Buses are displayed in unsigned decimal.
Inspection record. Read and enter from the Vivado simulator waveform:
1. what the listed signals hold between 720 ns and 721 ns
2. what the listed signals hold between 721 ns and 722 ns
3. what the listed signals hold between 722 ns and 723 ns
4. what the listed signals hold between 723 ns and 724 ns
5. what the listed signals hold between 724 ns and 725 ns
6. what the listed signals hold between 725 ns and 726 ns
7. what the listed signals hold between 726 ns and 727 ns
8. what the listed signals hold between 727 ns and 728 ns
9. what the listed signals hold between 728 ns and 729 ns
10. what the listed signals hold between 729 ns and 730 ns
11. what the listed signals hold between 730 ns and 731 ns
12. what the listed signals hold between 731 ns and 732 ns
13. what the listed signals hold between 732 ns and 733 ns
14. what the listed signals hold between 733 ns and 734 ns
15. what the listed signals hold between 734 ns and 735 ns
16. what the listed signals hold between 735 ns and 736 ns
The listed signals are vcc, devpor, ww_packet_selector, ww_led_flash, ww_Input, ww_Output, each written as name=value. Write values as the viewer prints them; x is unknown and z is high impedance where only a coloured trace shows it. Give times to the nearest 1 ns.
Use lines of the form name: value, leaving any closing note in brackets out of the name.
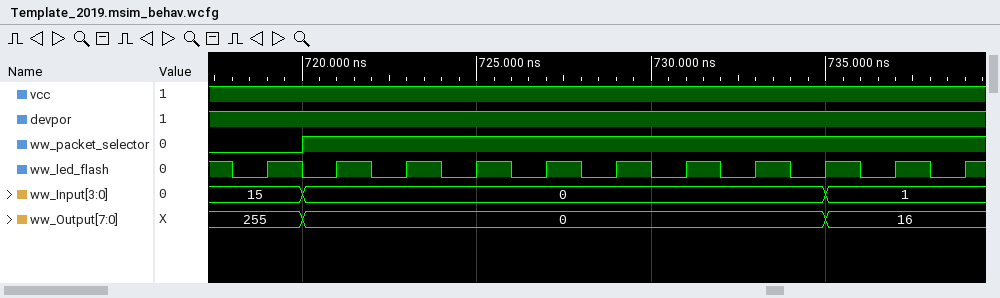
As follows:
what the listed signals hold between 720 ns and 721 ns: vcc=1, devpor=1, ww_packet_selector=1, ww_led_flash=0, ww_Input=0, ww_Output=0
what the listed signals hold between 721 ns and 722 ns: vcc=1, devpor=1, ww_packet_selector=1, ww_led_flash=1, ww_Input=0, ww_Output=0
what the listed signals hold between 722 ns and 723 ns: vcc=1, devpor=1, ww_packet_selector=1, ww_led_flash=0, ww_Input=0, ww_Output=0
what the listed signals hold between 723 ns and 724 ns: vcc=1, devpor=1, ww_packet_selector=1, ww_led_flash=1, ww_Input=0, ww_Output=0
what the listed signals hold between 724 ns and 725 ns: vcc=1, devpor=1, ww_packet_selector=1, ww_led_flash=0, ww_Input=0, ww_Output=0
what the listed signals hold between 725 ns and 726 ns: vcc=1, devpor=1, ww_packet_selector=1, ww_led_flash=1, ww_Input=0, ww_Output=0
what the listed signals hold between 726 ns and 727 ns: vcc=1, devpor=1, ww_packet_selector=1, ww_led_flash=0, ww_Input=0, ww_Output=0
what the listed signals hold between 727 ns and 728 ns: vcc=1, devpor=1, ww_packet_selector=1, ww_led_flash=1, ww_Input=0, ww_Output=0
what the listed signals hold between 728 ns and 729 ns: vcc=1, devpor=1, ww_packet_selector=1, ww_led_flash=0, ww_Input=0, ww_Output=0
what the listed signals hold between 729 ns and 730 ns: vcc=1, devpor=1, ww_packet_selector=1, ww_led_flash=1, ww_Input=0, ww_Output=0
what the listed signals hold between 730 ns and 731 ns: vcc=1, devpor=1, ww_packet_selector=1, ww_led_flash=0, ww_Input=0, ww_Output=0
what the listed signals hold between 731 ns and 732 ns: vcc=1, devpor=1, ww_packet_selector=1, ww_led_flash=1, ww_Input=0, ww_Output=0
what the listed signals hold between 732 ns and 733 ns: vcc=1, devpor=1, ww_packet_selector=1, ww_led_flash=0, ww_Input=0, ww_Output=0
what the listed signals hold between 733 ns and 734 ns: vcc=1, devpor=1, ww_packet_selector=1, ww_led_flash=1, ww_Input=0, ww_Output=0
what the listed signals hold between 734 ns and 735 ns: vcc=1, devpor=1, ww_packet_selector=1, ww_led_flash=0, ww_Input=0, ww_Output=0
what the listed signals hold between 735 ns and 736 ns: vcc=1, devpor=1, ww_packet_selector=1, ww_led_flash=1, ww_Input=1, ww_Output=16
